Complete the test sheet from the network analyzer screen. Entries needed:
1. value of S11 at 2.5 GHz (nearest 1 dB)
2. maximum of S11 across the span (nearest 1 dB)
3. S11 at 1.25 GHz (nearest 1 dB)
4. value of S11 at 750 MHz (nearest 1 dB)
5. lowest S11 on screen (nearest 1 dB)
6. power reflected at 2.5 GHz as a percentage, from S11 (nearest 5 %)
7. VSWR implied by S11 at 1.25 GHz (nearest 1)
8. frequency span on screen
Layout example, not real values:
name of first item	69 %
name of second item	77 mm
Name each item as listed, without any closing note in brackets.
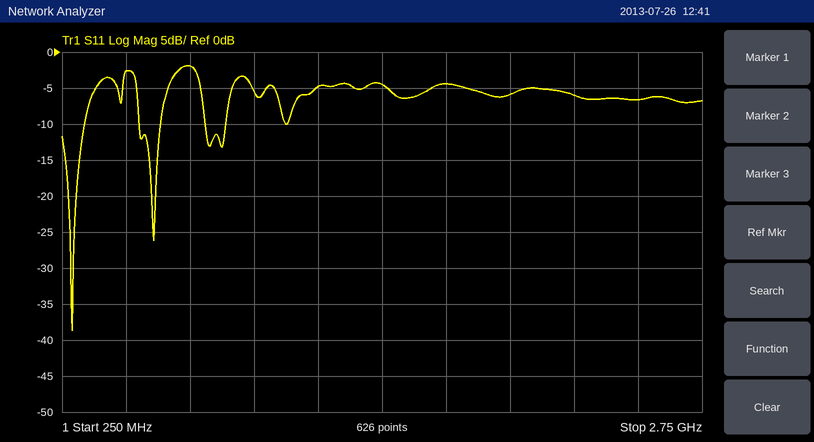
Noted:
value of S11 at 2.5 GHz	-7 dB
maximum of S11 across the span	-2 dB
S11 at 1.25 GHz	-5 dB
value of S11 at 750 MHz	-2 dB
lowest S11 on screen	-39 dB
power reflected at 2.5 GHz as a percentage, from S11	20 %
VSWR implied by S11 at 1.25 GHz	4
frequency span on screen	2.5 GHz
